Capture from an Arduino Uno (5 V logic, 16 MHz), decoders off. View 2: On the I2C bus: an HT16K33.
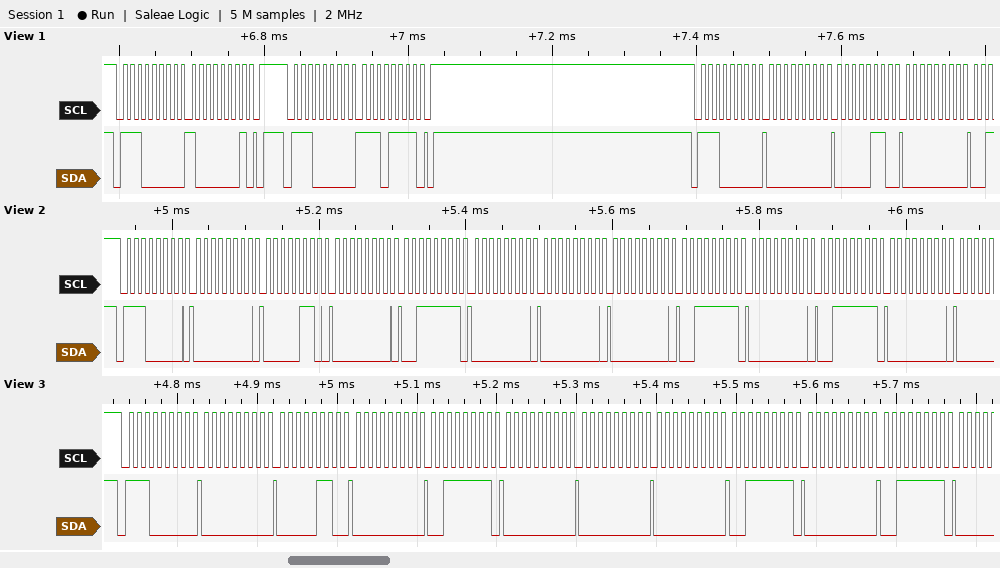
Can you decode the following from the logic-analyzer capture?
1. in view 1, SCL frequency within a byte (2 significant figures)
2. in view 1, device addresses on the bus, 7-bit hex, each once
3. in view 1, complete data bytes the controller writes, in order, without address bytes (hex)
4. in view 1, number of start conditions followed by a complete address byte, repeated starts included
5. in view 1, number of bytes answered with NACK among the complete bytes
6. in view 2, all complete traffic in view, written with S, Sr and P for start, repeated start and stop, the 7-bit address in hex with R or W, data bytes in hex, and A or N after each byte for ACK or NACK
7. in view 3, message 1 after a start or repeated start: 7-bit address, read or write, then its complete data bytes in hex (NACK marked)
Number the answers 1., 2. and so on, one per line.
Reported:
1. 100 kHz
2. 0x70
3. 81 EF 00 06 00
4. 3
5. 0
6. S 70W A 00 A 06 A 00 A 3F A 00 A 00 A 00 A 3F A 00 A 3F A 00 A
7. 0x70 write: 00 06 00 3F 00 00 00 3F 00 3F
